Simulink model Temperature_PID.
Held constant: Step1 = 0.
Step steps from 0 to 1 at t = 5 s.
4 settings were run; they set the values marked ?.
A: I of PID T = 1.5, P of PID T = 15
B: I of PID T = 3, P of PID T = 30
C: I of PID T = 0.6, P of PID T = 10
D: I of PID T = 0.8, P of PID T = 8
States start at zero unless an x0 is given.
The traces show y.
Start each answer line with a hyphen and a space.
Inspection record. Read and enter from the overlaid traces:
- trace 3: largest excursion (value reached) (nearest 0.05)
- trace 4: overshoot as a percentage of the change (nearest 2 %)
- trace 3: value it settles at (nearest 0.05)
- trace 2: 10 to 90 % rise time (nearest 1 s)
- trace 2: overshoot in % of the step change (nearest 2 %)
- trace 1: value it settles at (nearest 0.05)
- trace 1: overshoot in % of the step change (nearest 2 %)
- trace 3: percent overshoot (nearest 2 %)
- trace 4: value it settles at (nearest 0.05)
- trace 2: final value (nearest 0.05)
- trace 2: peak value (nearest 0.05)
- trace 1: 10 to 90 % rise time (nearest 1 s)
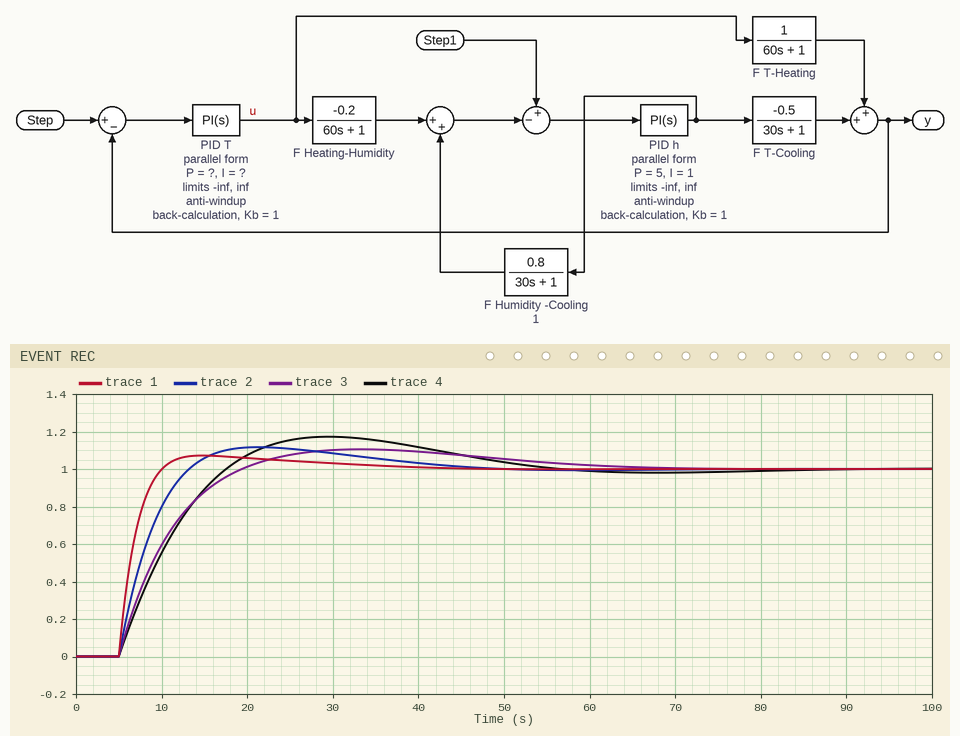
- 1.10
- 18 %
- 1.00
- 6 s
- 12 %
- 1.00
- 8 %
- 10 %
- 1.00
- 1.00
- 1.10
- 3 s
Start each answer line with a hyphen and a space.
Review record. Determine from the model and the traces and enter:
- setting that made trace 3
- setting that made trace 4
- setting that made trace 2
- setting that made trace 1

- C
- D
- A
- B
